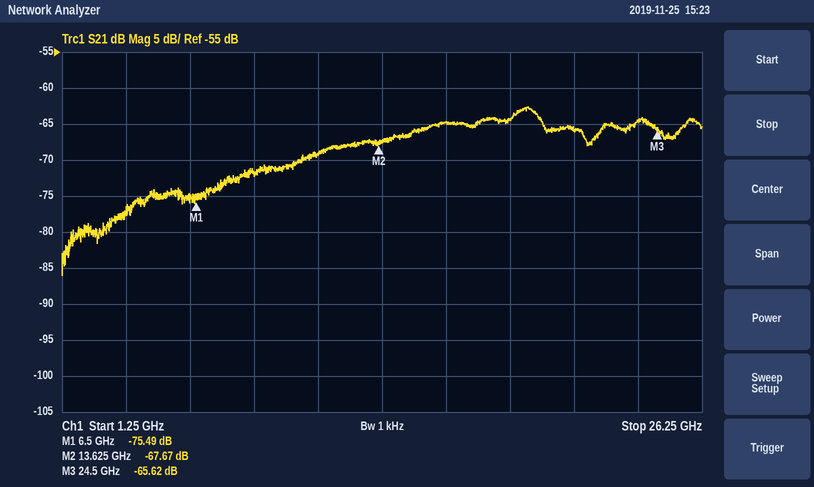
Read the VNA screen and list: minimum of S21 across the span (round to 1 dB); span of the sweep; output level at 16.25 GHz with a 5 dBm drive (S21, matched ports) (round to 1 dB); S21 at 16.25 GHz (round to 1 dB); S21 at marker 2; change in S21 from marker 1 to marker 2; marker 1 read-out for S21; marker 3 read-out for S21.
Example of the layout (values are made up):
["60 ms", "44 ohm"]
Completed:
["-86 dB", "25 GHz", "-60 dBm", "-65 dB", "-67.67 dB", "7.82 dB", "-75.49 dB", "-65.62 dB"]
